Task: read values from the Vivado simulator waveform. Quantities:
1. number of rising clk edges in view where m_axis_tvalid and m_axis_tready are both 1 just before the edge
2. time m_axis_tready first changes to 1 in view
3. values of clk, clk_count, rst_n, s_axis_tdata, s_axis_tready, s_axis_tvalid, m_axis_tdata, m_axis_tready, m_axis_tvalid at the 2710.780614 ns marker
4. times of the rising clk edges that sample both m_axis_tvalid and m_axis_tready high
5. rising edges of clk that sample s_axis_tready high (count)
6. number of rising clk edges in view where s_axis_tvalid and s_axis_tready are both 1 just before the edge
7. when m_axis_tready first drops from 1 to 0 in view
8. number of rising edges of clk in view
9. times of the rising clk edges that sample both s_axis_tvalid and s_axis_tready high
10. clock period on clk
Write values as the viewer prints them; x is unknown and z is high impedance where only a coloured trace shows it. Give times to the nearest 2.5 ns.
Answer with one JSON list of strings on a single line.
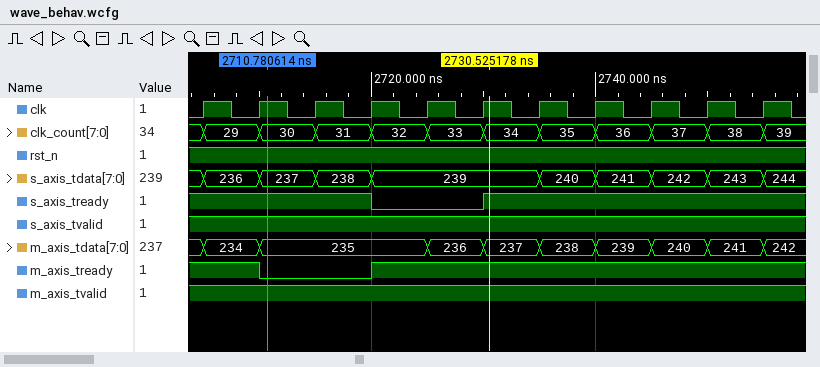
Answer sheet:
["9", "2720 ns", "clk=1, clk_count=30, rst_n=1, s_axis_tdata=237, s_axis_tready=1, s_axis_tvalid=1, m_axis_tdata=235, m_axis_tready=0, m_axis_tvalid=1", "2705 ns, 2710 ns, 2725 ns, 2730 ns, 2735 ns, 2740 ns, 2745 ns, 2750 ns, 2755 ns", "9", "9", "2710 ns", "11", "2705 ns, 2710 ns, 2715 ns, 2720 ns, 2735 ns, 2740 ns, 2745 ns, 2750 ns, 2755 ns", "5 ns"]
